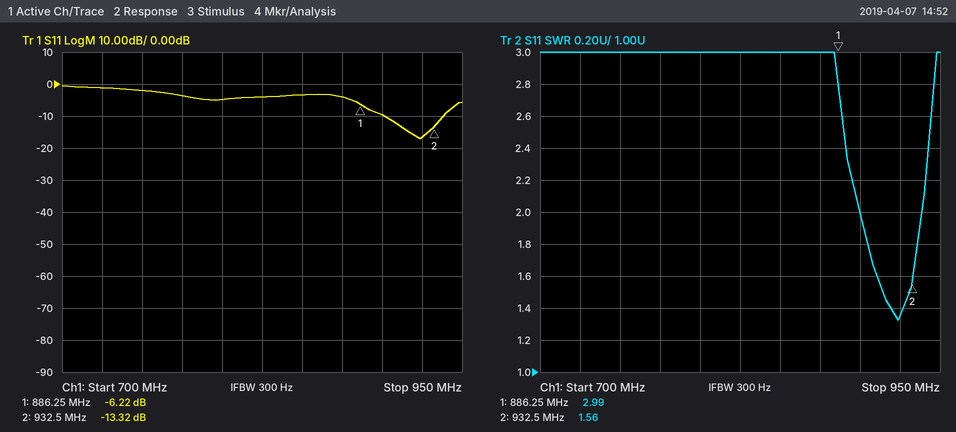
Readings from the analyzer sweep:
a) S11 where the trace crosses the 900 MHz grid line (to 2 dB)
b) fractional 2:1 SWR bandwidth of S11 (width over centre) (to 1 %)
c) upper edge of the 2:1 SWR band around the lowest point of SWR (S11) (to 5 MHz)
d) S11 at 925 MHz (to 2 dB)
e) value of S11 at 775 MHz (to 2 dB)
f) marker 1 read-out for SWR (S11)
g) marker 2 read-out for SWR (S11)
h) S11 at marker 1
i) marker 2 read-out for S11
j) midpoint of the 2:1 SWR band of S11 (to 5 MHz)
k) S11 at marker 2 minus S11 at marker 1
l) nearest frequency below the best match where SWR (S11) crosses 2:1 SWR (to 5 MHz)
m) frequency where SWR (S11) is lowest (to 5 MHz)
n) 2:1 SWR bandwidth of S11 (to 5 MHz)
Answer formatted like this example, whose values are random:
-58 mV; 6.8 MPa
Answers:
-10 dB; 4 %; 940 MHz; -16 dB; -4 dB; 2.99; 1.56; -6.22 dB; -13.32 dB; 920 MHz; -7.10 dB; 900 MHz; 925 MHz; 40 MHz
